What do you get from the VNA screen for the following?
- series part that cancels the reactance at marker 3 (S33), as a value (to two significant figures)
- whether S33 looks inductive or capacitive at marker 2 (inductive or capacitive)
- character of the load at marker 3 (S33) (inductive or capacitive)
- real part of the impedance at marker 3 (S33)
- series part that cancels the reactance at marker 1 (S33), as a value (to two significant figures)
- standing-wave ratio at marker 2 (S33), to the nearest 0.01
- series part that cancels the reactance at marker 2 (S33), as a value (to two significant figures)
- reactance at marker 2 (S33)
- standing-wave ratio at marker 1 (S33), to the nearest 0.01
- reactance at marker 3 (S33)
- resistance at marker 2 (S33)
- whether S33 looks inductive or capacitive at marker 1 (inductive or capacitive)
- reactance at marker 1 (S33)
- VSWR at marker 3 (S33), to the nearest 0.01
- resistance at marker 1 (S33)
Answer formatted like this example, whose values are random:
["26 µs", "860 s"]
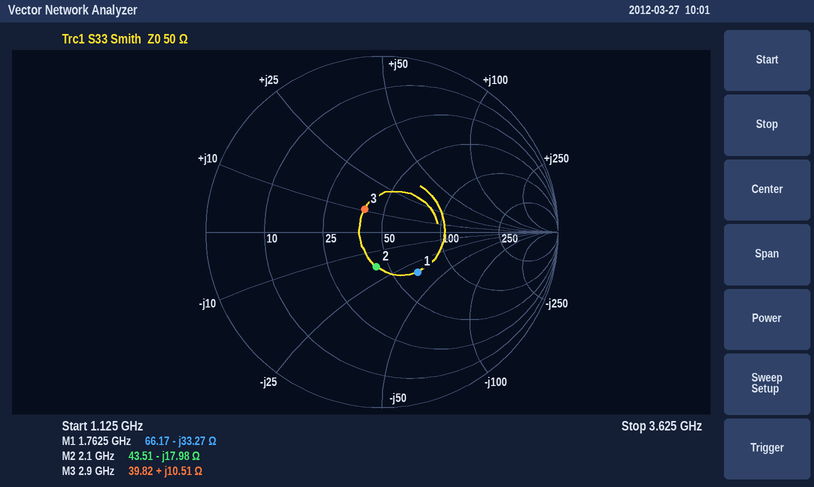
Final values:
["5.2 pF", "capacitive", "inductive", "39.82 Ω", "3.0 nH", "1.50", "1.4 nH", "-17.98 Ω", "1.88", "+10.51 Ω", "43.51 Ω", "capacitive", "-33.27 Ω", "1.39", "66.17 Ω"]
